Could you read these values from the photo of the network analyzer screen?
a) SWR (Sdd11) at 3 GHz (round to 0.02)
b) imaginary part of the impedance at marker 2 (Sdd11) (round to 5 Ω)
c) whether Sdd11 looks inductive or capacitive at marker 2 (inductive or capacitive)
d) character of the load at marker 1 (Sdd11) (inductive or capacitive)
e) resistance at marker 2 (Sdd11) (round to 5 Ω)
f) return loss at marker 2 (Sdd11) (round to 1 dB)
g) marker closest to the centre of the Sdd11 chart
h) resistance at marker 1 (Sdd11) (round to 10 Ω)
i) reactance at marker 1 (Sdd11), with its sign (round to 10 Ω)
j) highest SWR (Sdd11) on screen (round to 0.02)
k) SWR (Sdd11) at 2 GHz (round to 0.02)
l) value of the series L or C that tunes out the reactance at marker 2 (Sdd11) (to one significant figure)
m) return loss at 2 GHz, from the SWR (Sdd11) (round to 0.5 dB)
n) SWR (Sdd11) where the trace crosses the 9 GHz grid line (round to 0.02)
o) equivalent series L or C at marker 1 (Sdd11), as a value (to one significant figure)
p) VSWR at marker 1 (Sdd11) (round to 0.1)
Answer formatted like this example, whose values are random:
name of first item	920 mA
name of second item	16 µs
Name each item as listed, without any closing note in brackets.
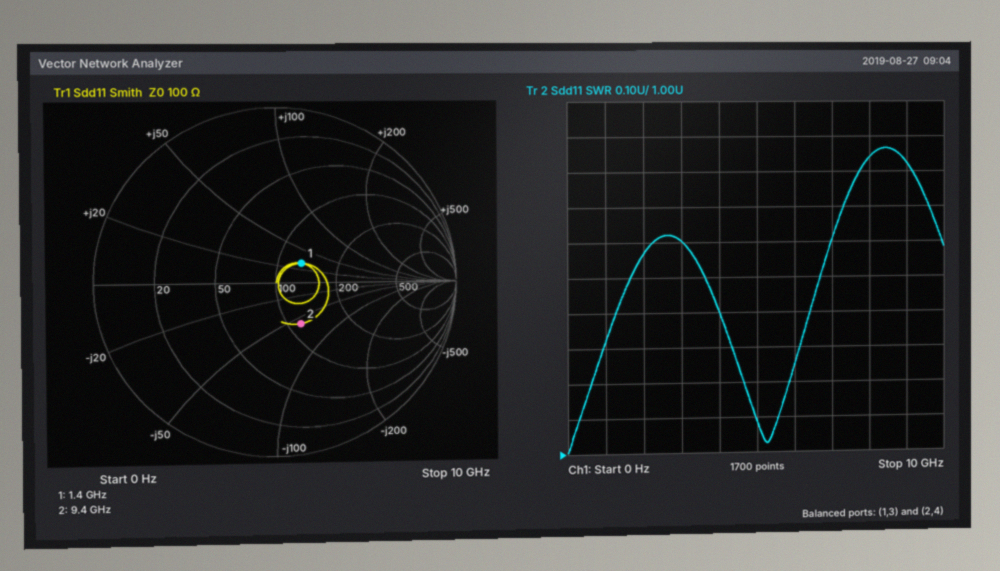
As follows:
SWR (Sdd11) at 3 GHz	1.60
imaginary part of the impedance at marker 2 (Sdd11)	-60 Ω
whether Sdd11 looks inductive or capacitive at marker 2	capacitive
character of the load at marker 1 (Sdd11)	inductive
resistance at marker 2 (Sdd11)	115 Ω
return loss at marker 2 (Sdd11)	11 dB
marker closest to the centre of the Sdd11 chart	marker 1
resistance at marker 1 (Sdd11)	130 Ω
reactance at marker 1 (Sdd11), with its sign	+30 Ω
highest SWR (Sdd11) on screen	1.86
SWR (Sdd11) at 2 GHz	1.56
value of the series L or C that tunes out the reactance at marker 2 (Sdd11)	1.0 nH
return loss at 2 GHz, from the SWR (Sdd11)	13.0 dB
SWR (Sdd11) where the trace crosses the 9 GHz grid line	1.82
equivalent series L or C at marker 1 (Sdd11), as a value	3 nH
VSWR at marker 1 (Sdd11)	1.4
